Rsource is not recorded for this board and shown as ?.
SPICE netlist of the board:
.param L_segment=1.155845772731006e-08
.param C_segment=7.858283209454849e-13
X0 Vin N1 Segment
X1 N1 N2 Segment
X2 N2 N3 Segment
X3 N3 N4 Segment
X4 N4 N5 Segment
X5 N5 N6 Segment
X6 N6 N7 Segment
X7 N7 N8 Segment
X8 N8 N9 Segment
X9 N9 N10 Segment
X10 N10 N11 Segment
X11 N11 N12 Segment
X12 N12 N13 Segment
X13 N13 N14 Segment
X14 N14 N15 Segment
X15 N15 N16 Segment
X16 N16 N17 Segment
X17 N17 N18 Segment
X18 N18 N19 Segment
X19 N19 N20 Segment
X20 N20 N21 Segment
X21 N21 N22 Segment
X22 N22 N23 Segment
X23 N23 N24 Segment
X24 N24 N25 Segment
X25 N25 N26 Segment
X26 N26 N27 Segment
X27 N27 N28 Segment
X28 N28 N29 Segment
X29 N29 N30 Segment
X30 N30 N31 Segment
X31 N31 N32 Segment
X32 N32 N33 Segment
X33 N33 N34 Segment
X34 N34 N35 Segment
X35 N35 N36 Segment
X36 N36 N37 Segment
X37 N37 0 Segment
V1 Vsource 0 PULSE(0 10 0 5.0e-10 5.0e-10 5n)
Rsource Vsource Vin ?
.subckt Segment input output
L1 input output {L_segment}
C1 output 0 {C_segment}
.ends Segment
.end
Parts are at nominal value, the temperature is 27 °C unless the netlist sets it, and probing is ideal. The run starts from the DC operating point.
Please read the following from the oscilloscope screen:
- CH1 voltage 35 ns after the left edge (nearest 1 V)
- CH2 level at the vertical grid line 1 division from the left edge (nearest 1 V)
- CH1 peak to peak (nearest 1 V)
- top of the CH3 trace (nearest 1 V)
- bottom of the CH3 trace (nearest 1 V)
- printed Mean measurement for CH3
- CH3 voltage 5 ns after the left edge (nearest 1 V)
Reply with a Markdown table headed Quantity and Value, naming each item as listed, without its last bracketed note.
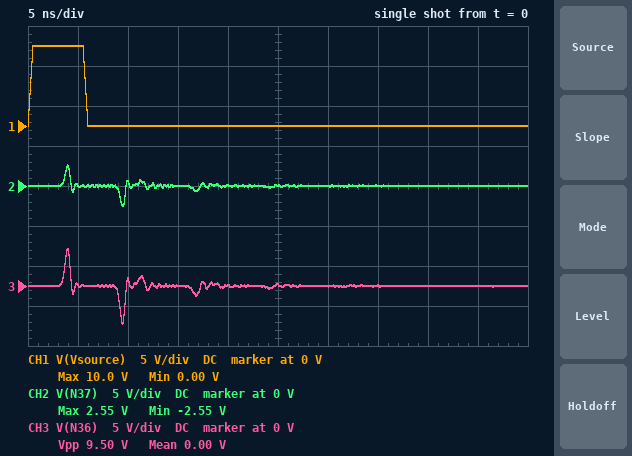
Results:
| Quantity | Value |
|---|---|
| CH1 voltage 35 ns after the left edge | 0 V |
| CH2 level at the vertical grid line 1 division from the left edge | 0 V |
| CH1 peak to peak | 10 V |
| top of the CH3 trace | 5 V |
| bottom of the CH3 trace | -5 V |
| printed Mean measurement for CH3 | 0.00 V |
| CH3 voltage 5 ns after the left edge | 0 V |
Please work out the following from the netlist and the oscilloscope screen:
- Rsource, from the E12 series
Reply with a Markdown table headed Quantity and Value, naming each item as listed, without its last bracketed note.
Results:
| Quantity | Value |
|---|---|
| Rsource, from the E12 series | 68 Ω |
